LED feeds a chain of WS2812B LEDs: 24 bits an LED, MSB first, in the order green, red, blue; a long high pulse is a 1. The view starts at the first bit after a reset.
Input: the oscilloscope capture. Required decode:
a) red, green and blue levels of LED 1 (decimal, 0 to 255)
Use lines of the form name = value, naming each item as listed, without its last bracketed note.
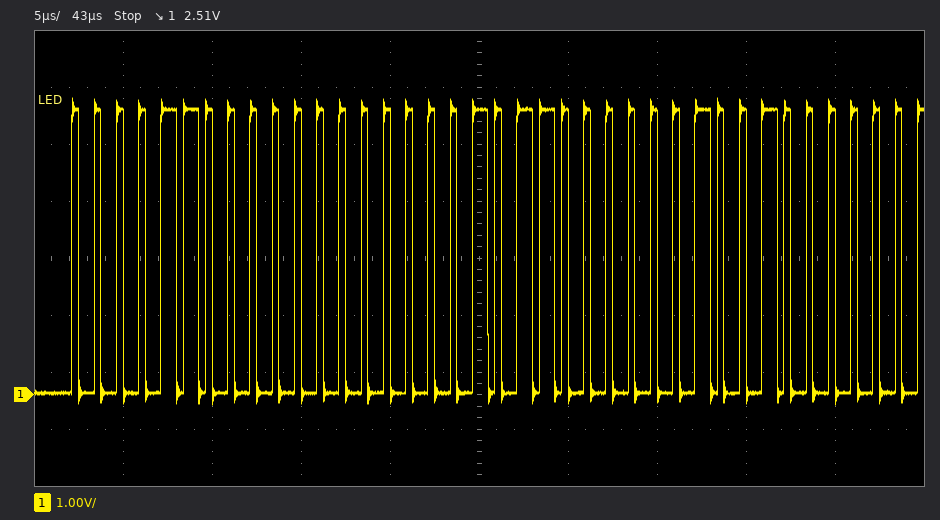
red, green and blue levels of LED 1 = 0, 12, 44
